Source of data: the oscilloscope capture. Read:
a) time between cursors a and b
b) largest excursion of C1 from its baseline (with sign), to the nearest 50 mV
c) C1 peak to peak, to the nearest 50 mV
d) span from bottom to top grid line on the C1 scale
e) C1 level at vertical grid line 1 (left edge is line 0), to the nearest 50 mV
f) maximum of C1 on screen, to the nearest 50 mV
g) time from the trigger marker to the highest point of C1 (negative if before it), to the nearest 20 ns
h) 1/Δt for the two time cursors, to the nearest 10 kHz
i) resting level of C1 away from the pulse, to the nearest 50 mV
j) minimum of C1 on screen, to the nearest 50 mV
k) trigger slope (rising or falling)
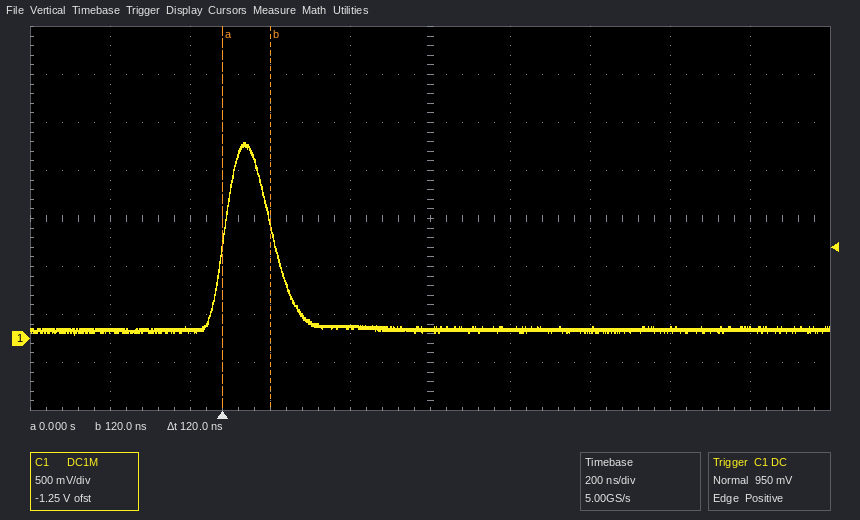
120 ns
+1.95 V
2.00 V
4 V
100 mV
2.05 V
+60 ns
8.33 MHz
100 mV
50 mV
rising
